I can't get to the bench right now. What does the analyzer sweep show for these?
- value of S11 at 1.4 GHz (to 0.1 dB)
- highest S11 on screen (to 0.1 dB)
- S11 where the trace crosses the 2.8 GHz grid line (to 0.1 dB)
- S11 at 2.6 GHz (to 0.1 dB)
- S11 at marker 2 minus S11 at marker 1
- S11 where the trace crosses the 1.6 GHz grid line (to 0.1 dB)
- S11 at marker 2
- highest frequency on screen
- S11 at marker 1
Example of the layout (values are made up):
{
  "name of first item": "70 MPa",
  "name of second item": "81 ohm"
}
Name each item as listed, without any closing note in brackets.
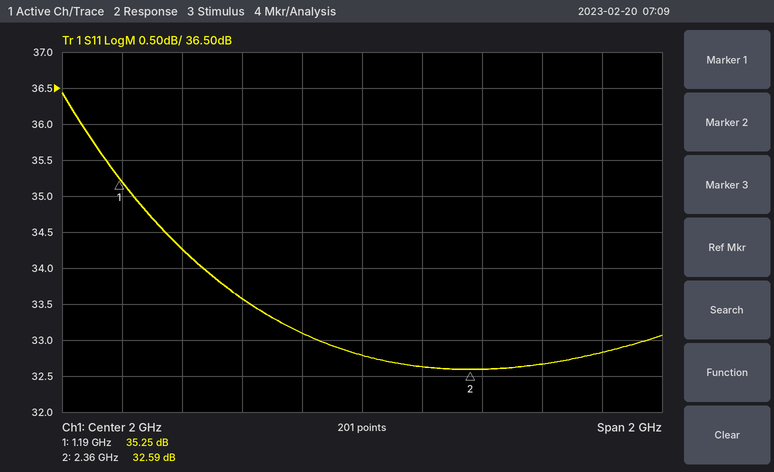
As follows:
{
  "value of S11 at 1.4 GHz": "34.3 dB",
  "highest S11 on screen": "36.4 dB",
  "S11 where the trace crosses the 2.8 GHz grid line": "32.8 dB",
  "S11 at 2.6 GHz": "32.7 dB",
  "S11 at marker 2 minus S11 at marker 1": "-2.66 dB",
  "S11 where the trace crosses the 1.6 GHz grid line": "33.6 dB",
  "S11 at marker 2": "32.59 dB",
  "highest frequency on screen": "3 GHz",
  "S11 at marker 1": "35.25 dB"
}
